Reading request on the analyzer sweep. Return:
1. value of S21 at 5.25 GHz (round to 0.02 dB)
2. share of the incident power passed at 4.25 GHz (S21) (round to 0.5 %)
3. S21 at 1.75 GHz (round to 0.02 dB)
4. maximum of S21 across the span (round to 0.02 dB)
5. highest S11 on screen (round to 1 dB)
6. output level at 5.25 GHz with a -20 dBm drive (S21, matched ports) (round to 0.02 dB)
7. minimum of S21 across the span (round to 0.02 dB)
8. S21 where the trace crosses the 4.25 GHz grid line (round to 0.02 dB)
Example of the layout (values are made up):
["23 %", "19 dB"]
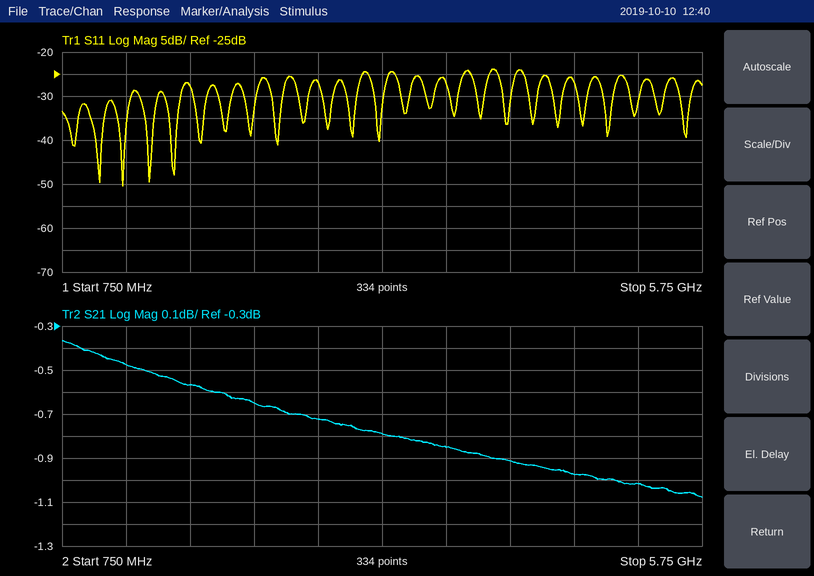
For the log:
["-1.02 dB", "81.0 %", "-0.56 dB", "-0.36 dB", "-24 dB", "-21.02 dBm", "-1.08 dB", "-0.92 dB"]
